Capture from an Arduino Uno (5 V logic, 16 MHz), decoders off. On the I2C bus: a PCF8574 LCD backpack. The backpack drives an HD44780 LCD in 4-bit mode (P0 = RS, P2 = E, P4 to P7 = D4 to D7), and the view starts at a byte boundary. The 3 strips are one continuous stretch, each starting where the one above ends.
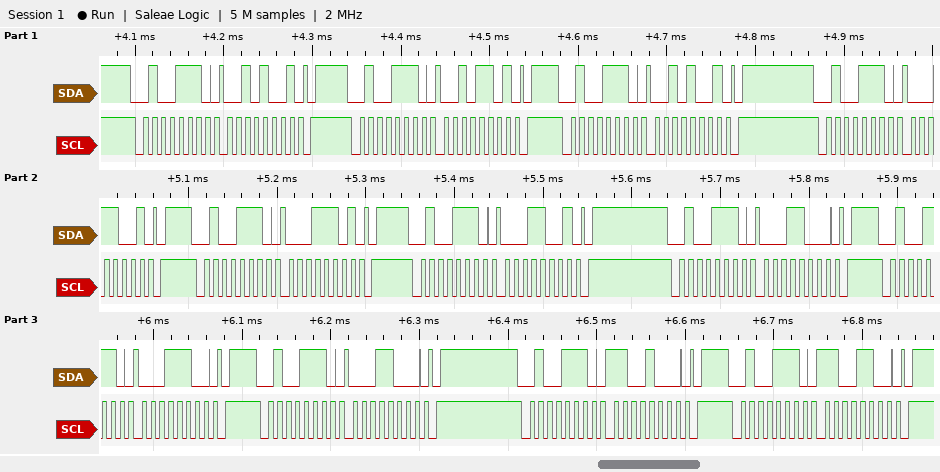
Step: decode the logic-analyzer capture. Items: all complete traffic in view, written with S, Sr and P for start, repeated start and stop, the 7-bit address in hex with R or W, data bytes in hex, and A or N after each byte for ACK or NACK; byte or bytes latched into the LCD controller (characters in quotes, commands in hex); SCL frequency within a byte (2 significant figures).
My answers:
S 27W A 29 A P S 27W A 2D A P S 27W A 29 A P S 27W A 19 A P S 27W A 1D A P S 27W A 19 A P S 27W A 18 A P S 27W A 1C A P S 27W A 18 A P S 27W A C8 A P S 27W A CC A P
'!'
100 kHz
